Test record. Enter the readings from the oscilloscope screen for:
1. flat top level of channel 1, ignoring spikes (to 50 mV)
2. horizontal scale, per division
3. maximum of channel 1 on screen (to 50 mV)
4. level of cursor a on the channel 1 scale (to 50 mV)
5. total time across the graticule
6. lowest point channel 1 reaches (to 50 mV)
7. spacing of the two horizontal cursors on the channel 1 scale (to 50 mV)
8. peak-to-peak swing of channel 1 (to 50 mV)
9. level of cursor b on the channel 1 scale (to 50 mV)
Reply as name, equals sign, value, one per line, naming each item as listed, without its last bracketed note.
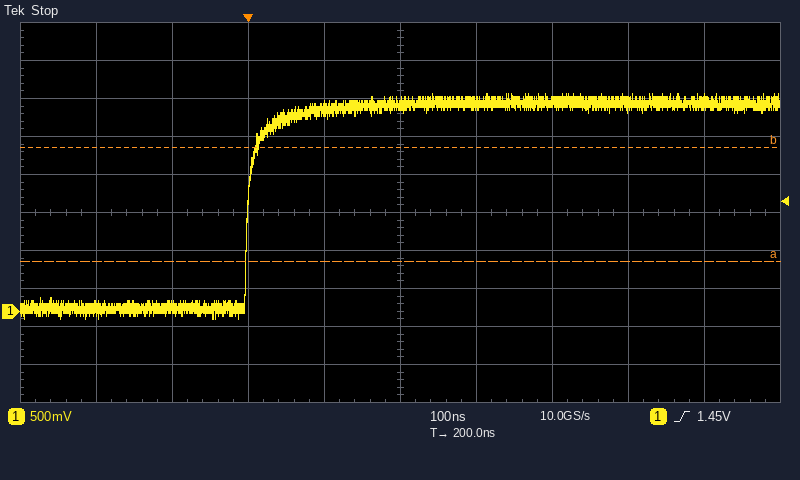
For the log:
flat top level of channel 1, ignoring spikes = 2.75 V
horizontal scale, per division = 100 ns
maximum of channel 1 on screen = 2.85 V
level of cursor a on the channel 1 scale = 650 mV
total time across the graticule = 1 µs
lowest point channel 1 reaches = -100 mV
spacing of the two horizontal cursors on the channel 1 scale = 1.50 V
peak-to-peak swing of channel 1 = 2.95 V
level of cursor b on the channel 1 scale = 2.15 V
